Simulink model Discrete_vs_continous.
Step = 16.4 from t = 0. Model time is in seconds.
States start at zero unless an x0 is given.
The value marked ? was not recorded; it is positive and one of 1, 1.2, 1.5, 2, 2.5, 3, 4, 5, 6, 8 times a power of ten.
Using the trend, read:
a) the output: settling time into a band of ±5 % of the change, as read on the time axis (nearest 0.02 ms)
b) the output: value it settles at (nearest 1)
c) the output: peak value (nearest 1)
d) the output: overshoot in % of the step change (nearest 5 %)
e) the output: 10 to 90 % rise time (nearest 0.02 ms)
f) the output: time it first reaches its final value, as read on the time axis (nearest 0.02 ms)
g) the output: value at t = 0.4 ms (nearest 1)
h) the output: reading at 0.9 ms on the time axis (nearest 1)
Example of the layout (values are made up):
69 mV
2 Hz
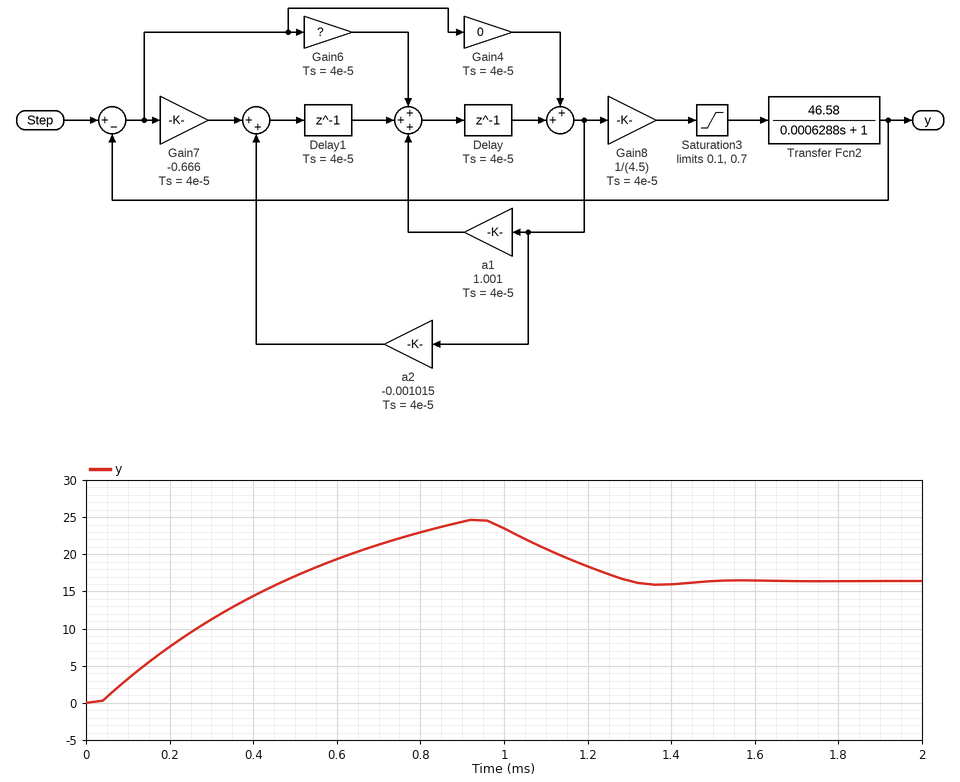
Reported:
1.26 ms
16
25
50 %
0.34 ms
0.48 ms
14
24
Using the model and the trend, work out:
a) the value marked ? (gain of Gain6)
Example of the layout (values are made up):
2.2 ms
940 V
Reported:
0.8
